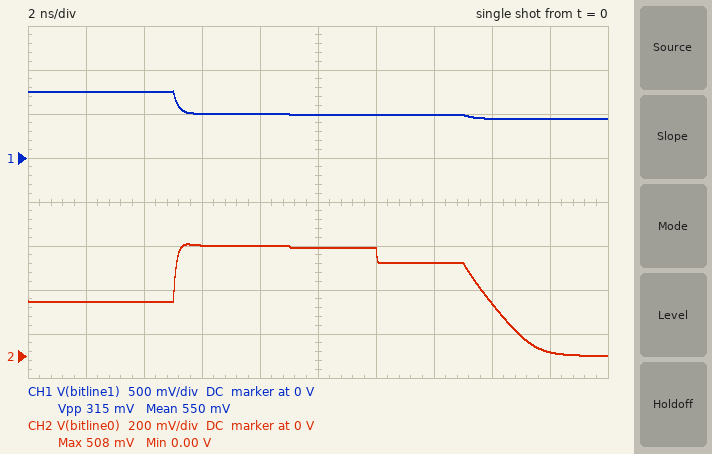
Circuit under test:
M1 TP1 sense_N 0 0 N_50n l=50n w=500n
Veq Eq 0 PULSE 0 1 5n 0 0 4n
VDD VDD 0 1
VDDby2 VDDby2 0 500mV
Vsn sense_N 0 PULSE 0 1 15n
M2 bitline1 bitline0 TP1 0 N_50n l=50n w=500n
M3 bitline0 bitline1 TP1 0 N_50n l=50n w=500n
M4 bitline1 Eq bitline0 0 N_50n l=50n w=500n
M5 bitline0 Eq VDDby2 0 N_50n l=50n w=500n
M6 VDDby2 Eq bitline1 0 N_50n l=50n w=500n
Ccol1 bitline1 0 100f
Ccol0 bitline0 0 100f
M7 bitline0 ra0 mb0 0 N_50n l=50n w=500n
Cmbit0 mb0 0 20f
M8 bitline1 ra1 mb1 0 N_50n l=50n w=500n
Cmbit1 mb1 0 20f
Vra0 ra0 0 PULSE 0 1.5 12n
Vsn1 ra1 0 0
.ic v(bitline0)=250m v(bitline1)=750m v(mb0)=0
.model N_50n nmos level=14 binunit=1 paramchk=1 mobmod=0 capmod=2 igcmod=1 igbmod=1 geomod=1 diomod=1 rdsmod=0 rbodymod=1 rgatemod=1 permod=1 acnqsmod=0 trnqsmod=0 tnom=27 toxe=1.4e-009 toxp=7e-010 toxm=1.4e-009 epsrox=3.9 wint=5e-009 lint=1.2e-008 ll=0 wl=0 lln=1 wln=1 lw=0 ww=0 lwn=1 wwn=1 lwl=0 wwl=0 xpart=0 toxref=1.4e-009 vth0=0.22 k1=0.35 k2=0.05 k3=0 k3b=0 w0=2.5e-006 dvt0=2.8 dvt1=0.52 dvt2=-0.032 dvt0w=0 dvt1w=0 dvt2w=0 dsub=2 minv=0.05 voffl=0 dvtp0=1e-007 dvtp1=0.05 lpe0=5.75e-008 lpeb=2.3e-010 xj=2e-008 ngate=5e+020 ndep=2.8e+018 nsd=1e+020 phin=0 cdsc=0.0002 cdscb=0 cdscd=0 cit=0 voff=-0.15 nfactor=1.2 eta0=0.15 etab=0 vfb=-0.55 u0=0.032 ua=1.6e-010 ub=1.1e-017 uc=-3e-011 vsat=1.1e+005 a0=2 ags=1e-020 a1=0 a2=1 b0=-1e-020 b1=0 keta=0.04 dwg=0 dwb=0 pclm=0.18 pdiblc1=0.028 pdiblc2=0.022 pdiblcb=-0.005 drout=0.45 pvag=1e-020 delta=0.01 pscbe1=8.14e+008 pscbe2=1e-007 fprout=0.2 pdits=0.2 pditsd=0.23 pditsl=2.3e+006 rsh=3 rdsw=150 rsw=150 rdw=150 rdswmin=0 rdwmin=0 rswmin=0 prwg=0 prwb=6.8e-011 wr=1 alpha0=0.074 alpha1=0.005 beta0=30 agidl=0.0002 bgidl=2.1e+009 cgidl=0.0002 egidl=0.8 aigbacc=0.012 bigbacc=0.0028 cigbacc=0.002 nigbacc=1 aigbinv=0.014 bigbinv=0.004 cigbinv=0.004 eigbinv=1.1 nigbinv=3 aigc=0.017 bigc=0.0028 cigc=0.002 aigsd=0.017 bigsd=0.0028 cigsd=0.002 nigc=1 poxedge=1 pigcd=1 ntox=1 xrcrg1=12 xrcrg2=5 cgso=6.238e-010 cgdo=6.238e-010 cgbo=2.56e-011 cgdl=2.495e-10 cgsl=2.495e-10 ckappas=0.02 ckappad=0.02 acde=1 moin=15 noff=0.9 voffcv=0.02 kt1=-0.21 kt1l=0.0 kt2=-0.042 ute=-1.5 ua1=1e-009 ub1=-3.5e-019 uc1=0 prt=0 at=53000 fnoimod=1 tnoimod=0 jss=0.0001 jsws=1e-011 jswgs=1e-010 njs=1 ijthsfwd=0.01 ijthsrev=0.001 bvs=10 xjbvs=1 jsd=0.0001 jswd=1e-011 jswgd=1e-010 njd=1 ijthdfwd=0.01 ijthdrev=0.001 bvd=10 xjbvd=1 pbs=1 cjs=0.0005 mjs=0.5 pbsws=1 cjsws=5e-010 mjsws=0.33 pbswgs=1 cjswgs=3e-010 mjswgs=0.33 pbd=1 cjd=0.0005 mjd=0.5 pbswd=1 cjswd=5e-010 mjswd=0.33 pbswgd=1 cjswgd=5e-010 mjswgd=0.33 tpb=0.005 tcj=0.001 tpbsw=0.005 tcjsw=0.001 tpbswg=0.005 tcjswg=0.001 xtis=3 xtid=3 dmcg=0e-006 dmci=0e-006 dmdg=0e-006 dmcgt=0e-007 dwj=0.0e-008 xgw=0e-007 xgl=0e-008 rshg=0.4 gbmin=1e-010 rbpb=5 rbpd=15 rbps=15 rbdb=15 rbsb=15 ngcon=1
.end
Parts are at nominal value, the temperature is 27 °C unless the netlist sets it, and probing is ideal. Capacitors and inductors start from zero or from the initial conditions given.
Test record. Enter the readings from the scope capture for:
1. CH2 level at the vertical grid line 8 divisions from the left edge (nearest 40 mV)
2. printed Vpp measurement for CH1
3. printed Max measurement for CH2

240 mV
315 mV
508 mV
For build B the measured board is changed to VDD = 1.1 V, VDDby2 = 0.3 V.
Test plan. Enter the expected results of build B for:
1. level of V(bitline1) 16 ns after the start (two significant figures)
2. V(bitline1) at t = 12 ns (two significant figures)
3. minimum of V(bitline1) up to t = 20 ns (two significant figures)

280 mV
290 mV
260 mV
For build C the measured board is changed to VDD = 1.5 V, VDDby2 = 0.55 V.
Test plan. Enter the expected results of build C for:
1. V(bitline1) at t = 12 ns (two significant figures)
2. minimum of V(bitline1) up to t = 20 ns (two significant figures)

540 mV
490 mV
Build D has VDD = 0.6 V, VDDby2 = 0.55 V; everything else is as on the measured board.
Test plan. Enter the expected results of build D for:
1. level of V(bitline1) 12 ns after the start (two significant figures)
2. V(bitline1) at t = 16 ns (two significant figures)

540 mV
490 mV
